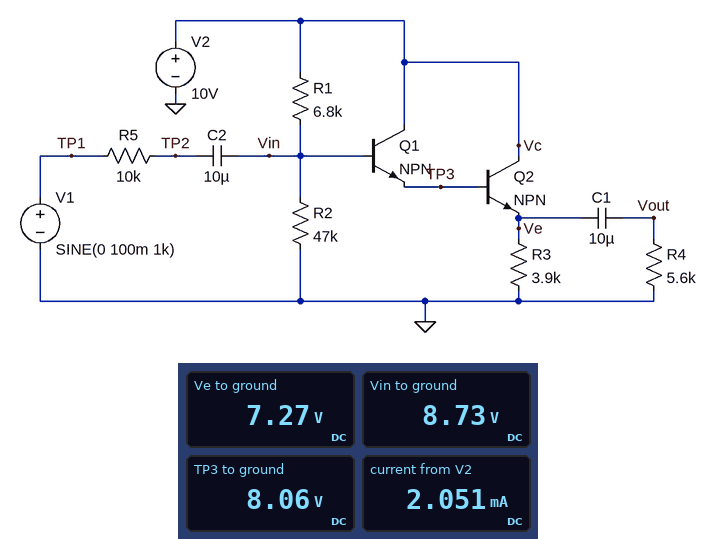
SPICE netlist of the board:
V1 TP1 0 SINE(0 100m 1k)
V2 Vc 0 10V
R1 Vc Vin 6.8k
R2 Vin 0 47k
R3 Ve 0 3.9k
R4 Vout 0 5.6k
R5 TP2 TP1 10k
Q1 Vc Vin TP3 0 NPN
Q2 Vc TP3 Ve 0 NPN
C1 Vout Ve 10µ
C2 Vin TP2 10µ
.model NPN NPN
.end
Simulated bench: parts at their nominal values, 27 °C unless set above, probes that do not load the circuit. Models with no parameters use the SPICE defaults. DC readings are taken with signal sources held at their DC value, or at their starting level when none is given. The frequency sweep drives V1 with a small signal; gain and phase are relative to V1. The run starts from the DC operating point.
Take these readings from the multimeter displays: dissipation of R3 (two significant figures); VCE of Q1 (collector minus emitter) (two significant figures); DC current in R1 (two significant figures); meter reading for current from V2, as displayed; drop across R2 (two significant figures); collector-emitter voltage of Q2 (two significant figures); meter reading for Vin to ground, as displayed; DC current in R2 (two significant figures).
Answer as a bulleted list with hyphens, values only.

- 14 mW
- 1.9 V
- 190 µA
- 2.051 mA
- 8.7 V
- 2.7 V
- 8.73 V
- 190 µA
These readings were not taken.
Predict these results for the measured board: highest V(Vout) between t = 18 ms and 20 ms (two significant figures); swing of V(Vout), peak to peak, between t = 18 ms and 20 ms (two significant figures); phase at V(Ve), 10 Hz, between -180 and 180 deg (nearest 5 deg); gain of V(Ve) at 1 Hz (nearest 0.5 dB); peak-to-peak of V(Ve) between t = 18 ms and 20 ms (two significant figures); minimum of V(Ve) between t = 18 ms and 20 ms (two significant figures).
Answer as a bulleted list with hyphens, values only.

- 37 mV
- 74 mV
- 5 deg
- -11.5 dB
- 74 mV
- 7.2 V
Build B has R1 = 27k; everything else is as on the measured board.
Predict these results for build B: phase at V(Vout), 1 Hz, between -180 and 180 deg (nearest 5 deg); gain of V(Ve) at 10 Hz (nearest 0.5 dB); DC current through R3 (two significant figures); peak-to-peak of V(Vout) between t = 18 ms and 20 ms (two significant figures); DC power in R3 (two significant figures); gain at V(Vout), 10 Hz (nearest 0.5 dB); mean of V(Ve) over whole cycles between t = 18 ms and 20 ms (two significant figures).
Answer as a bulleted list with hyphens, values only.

- 100 deg
- -4.0 dB
- 1.3 mA
- 120 mV
- 6.2 mW
- -4.5 dB
- 4.9 V
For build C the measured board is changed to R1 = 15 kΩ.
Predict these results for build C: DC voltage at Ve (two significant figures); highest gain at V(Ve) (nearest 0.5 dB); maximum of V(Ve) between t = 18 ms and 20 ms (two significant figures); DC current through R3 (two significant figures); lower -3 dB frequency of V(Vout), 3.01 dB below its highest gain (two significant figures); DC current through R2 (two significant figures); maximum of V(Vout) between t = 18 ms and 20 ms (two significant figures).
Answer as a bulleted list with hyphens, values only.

- 6.1 V
- -5.5 dB
- 6.2 V
- 1.6 mA
- 3.0 Hz
- 160 µA
- 52 mV
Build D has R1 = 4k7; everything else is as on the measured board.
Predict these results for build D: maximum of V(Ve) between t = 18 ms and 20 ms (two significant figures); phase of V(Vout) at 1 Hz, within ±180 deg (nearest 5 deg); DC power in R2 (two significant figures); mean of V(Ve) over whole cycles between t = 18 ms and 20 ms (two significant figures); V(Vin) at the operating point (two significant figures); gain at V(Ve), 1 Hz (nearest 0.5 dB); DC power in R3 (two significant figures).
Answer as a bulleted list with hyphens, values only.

- 7.7 V
- 120 deg
- 1.8 mW
- 7.6 V
- 9.1 V
- -14.0 dB
- 15 mW
